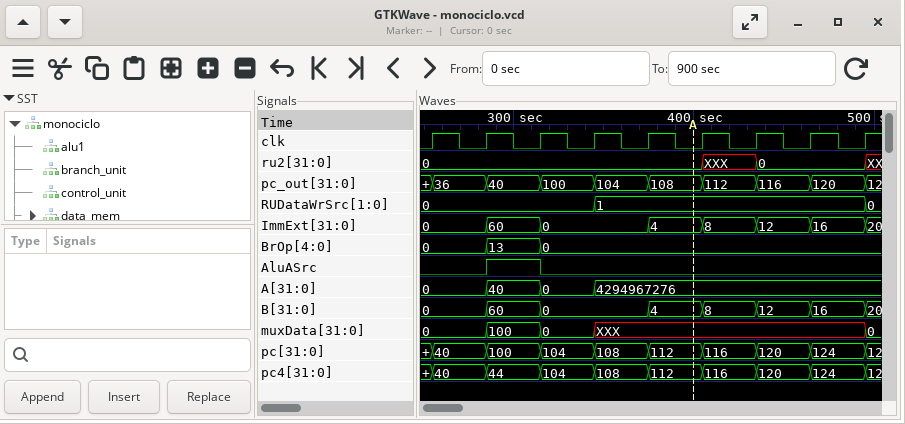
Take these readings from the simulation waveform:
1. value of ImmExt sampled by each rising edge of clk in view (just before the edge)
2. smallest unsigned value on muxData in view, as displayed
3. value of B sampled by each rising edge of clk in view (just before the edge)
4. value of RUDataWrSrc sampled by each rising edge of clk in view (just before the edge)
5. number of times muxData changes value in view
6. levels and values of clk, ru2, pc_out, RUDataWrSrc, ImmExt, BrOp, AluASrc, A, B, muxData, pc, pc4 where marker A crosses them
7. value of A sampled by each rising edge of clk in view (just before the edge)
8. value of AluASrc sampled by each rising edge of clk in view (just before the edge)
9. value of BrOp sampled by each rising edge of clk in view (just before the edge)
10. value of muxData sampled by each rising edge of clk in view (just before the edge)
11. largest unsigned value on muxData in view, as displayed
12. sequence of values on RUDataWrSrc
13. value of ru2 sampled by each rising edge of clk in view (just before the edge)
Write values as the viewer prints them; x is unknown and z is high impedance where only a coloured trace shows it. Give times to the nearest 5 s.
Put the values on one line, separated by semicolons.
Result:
0, 0, 60, 0, 0, 4, 8, 12, 16; 0; 0, 0, 60, 0, 0, 4, 8, 12, 16; 0, 0, 0, 0, 1, 1, 1, 1, 1; 4; clk=0, ru2=0, pc_out=108, RUDataWrSrc=1, ImmExt=4, BrOp=0, AluASrc=0, A=4294967276, B=4, muxData=XXX, pc=112, pc4=112; 0, 0, 40, 0, 4294967276, 4294967276, 4294967276, 4294967276, 4294967276; 0 0 1 0 0 0 0 0 0; 0, 0, 13, 0, 0, 0, 0, 0, 0; 0, 0, 100, 0, XXX, XXX, XXX, XXX, XXX; 100; 0, 1, 0; 0, 0, 0, 0, 0, 0, XXX, 0, 0
